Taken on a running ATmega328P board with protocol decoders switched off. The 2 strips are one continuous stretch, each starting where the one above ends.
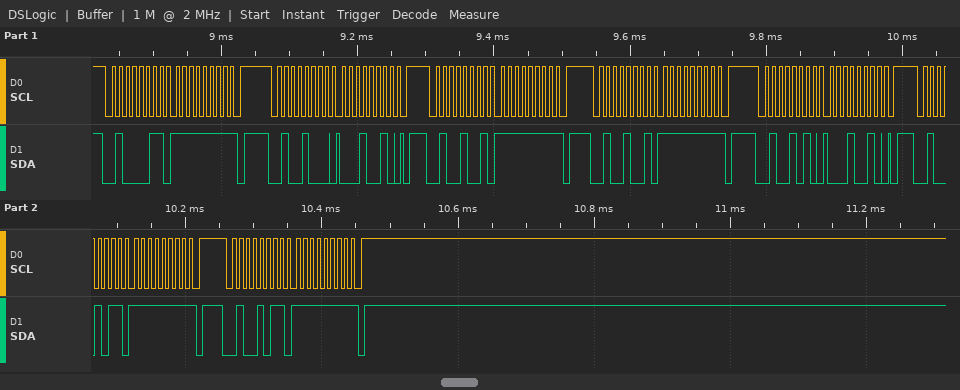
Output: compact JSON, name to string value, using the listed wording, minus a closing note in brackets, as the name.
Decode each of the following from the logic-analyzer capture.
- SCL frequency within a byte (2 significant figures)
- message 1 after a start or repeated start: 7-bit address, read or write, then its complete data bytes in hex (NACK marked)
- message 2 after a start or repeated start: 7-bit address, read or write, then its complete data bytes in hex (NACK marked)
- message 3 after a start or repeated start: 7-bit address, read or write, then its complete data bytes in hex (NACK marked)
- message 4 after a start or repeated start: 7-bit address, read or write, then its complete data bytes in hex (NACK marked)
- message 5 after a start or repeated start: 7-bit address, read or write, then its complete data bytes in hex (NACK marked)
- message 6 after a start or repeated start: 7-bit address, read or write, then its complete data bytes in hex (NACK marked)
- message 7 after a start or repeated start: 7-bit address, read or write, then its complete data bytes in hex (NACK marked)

{"SCL frequency within a byte": "100 kHz", "message 1 after a start or repeated start: 7-bit address, read or write, then its complete data bytes in hex": "0x21 read: FF NACK", "message 2 after a start or repeated start: 7-bit address, read or write, then its complete data bytes in hex": "0x24 write: 12", "message 3 after a start or repeated start: 7-bit address, read or write, then its complete data bytes in hex": "0x24 read: FF NACK", "message 4 after a start or repeated start: 7-bit address, read or write, then its complete data bytes in hex": "0x24 read: FF NACK", "message 5 after a start or repeated start: 7-bit address, read or write, then its complete data bytes in hex": "0x25 write: 12", "message 6 after a start or repeated start: 7-bit address, read or write, then its complete data bytes in hex": "0x25 read: FF NACK", "message 7 after a start or repeated start: 7-bit address, read or write, then its complete data bytes in hex": "0x25 read: FF NACK"}
